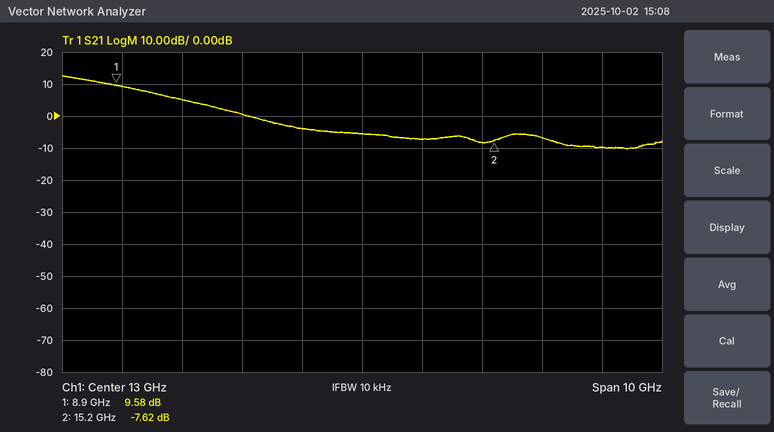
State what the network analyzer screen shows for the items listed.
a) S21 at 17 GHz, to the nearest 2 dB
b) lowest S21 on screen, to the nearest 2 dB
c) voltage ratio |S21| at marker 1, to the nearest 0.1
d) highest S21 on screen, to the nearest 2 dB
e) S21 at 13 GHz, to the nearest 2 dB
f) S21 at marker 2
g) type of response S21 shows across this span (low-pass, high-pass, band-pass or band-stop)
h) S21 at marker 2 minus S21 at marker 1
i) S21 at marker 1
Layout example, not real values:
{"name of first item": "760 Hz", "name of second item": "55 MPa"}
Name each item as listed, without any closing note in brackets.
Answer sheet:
{"S21 at 17 GHz, to the nearest 2 dB": "-10 dB", "lowest S21 on screen, to the nearest 2 dB": "-10 dB", "voltage ratio |S21| at marker 1, to the nearest 0.1": "3.0", "highest S21 on screen, to the nearest 2 dB": "12 dB", "S21 at 13 GHz, to the nearest 2 dB": "-6 dB", "S21 at marker 2": "-7.62 dB", "type of response S21 shows across this span": "low-pass", "S21 at marker 2 minus S21 at marker 1": "-17.20 dB", "S21 at marker 1": "9.58 dB"}
